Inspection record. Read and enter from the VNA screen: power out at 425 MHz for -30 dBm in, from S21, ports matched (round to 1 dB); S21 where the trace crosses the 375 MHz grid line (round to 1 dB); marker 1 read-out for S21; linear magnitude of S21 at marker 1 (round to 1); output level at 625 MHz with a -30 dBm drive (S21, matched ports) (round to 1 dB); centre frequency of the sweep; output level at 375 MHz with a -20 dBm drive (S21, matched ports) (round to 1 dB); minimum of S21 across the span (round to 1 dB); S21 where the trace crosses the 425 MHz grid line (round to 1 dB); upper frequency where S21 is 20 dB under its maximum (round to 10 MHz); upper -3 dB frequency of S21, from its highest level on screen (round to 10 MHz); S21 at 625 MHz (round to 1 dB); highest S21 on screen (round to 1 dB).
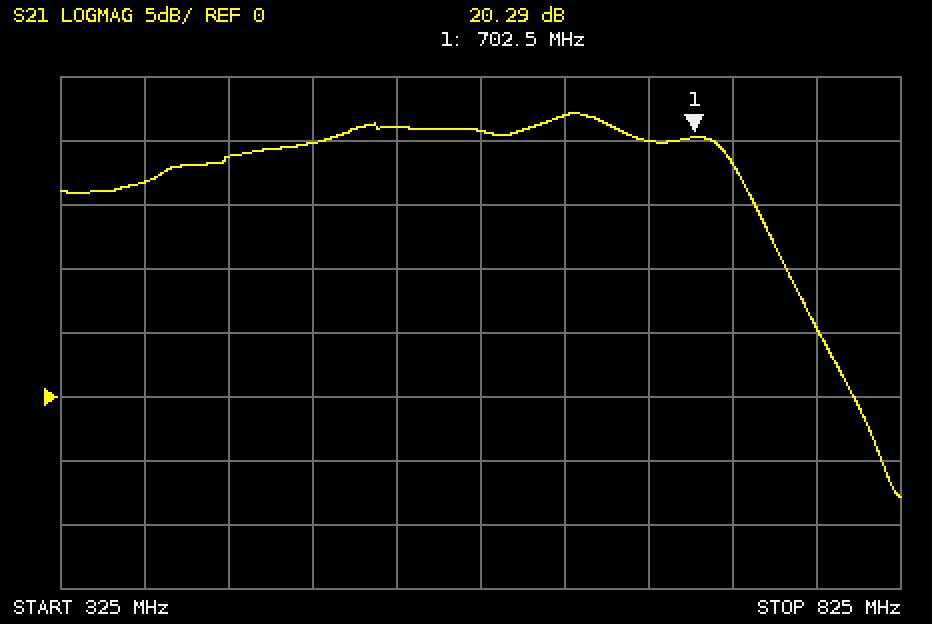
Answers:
-11 dBm
17 dB
20.29 dB
10
-8 dBm
575 MHz
-3 dBm
-8 dB
19 dB
790 MHz
720 MHz
22 dB
22 dB
